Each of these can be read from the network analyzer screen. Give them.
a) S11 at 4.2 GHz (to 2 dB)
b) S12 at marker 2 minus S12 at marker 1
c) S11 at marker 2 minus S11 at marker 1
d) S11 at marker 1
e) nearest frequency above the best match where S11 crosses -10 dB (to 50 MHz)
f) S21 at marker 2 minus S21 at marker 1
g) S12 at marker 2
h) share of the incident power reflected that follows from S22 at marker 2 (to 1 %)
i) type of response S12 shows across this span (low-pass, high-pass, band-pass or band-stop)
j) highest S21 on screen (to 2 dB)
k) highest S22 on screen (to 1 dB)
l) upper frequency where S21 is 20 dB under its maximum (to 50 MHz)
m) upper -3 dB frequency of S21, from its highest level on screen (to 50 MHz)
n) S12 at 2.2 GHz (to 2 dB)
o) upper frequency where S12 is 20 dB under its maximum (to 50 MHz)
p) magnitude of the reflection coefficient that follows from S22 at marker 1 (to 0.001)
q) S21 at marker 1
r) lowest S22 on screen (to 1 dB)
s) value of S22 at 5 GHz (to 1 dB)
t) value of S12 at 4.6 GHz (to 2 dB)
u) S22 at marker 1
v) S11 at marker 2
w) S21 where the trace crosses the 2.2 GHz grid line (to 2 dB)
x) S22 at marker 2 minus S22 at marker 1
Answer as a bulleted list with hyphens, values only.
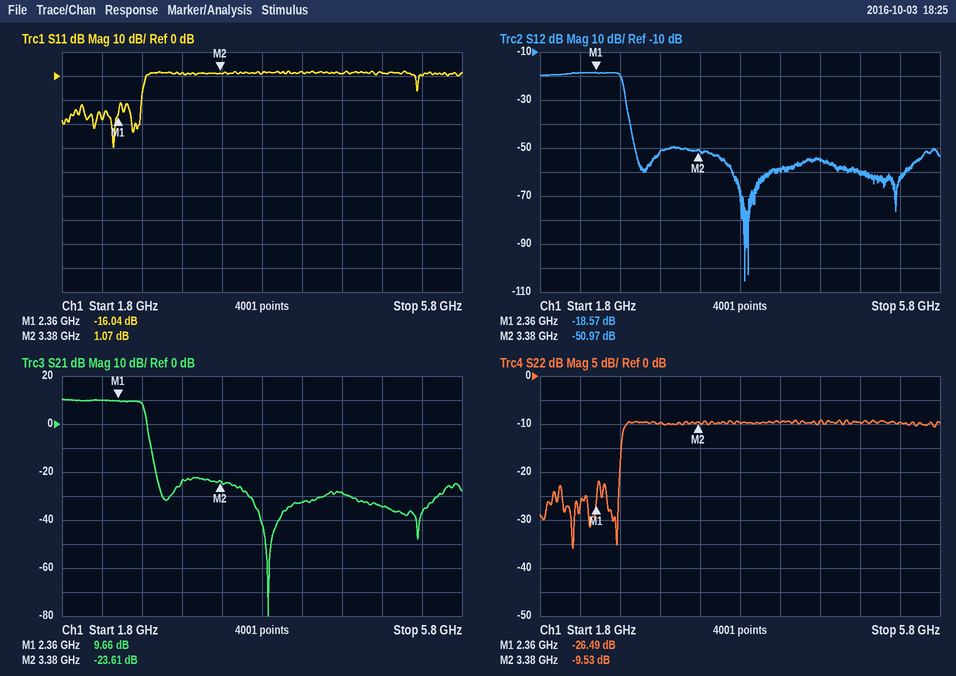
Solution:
- 2 dB
- -32.40 dB
- 17.11 dB
- -16.04 dB
- 2.60 GHz
- -33.27 dB
- -50.97 dB
- 11 %
- low-pass
- 10 dB
- -9 dB
- 2.70 GHz
- 2.60 GHz
- -18 dB
- 2.70 GHz
- 0.047
- 9.66 dB
- -36 dB
- -10 dB
- -54 dB
- -26.49 dB
- 1.07 dB
- 10 dB
- 16.96 dB
